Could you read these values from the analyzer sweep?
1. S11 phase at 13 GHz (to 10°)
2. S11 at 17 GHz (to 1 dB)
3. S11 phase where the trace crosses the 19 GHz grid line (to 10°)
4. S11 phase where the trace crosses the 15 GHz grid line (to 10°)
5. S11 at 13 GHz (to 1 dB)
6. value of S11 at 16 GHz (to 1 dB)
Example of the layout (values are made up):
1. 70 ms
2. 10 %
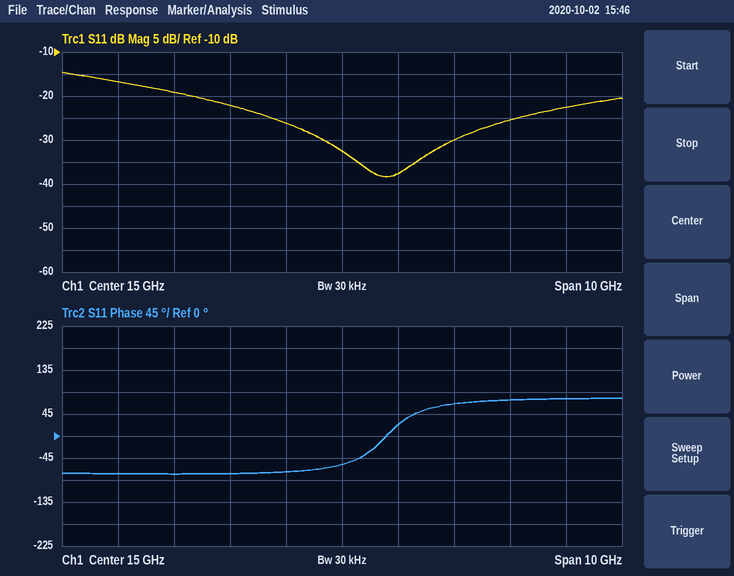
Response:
1. -80°
2. -30 dB
3. 80°
4. -60°
5. -22 dB
6. -38 dB
